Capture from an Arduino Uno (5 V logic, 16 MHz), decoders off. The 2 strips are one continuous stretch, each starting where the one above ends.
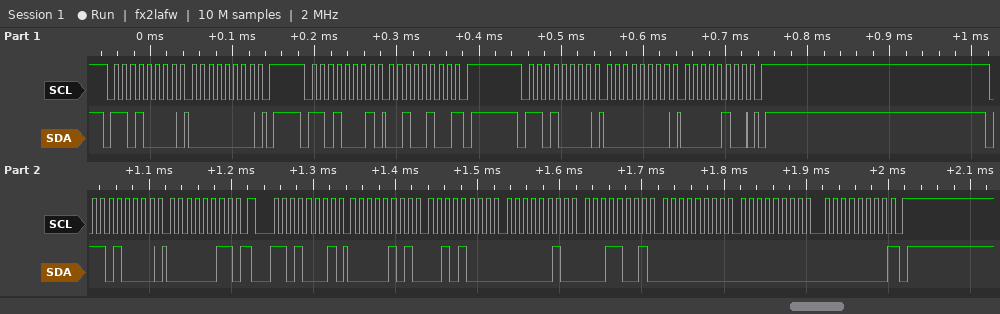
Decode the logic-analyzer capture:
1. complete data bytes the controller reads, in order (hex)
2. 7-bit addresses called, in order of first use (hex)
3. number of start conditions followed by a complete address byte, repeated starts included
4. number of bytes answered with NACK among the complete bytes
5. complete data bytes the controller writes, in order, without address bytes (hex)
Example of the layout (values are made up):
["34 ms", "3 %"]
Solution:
["24 05 28 02 19 00 00 00", "0x68", "5", "2", "00 00 04 03"]
